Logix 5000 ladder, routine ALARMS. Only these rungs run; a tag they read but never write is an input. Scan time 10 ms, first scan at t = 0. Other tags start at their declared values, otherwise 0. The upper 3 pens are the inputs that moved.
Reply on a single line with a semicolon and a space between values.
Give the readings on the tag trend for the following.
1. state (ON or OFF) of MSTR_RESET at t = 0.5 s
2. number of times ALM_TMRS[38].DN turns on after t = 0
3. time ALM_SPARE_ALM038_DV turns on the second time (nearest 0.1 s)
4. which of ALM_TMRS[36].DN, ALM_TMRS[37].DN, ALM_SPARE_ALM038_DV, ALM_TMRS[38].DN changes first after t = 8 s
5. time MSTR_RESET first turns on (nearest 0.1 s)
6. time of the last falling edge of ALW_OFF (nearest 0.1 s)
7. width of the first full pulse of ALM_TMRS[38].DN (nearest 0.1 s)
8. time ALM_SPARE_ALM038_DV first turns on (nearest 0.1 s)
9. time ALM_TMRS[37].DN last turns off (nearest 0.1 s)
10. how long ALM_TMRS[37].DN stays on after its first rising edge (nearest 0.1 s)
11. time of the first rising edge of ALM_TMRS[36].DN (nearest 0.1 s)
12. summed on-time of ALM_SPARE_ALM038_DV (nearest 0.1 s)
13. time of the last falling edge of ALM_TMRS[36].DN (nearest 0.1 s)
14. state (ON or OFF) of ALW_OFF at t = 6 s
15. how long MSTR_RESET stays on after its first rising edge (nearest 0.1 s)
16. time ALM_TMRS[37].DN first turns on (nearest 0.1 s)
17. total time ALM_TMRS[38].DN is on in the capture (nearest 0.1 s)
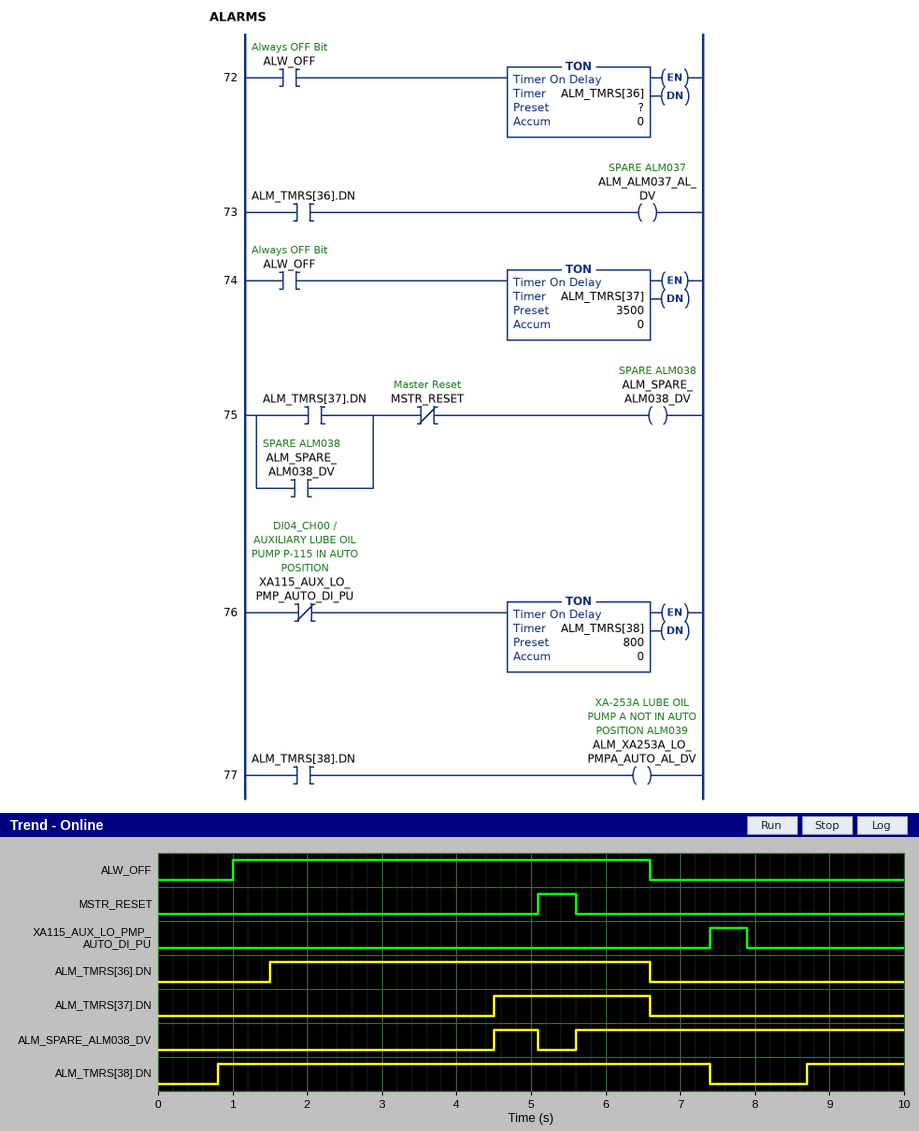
OFF; 2; 5.6 s; ALM_TMRS[38].DN; 5.1 s; 6.6 s; 6.6 s; 4.5 s; 6.6 s; 2.1 s; 1.5 s; 5.0 s; 6.6 s; ON; 0.5 s; 4.5 s; 7.9 s
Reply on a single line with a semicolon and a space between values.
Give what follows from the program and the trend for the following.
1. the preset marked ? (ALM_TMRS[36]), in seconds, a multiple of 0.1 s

0.5 s
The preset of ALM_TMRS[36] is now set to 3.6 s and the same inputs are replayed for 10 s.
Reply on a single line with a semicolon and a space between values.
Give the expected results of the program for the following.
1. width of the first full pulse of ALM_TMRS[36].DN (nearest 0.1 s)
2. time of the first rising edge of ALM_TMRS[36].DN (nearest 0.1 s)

2.0 s; 4.6 s
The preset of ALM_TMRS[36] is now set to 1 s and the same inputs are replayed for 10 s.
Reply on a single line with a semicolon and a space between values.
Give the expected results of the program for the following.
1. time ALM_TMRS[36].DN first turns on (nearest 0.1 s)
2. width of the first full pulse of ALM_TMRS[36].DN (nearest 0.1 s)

2.0 s; 4.6 s
